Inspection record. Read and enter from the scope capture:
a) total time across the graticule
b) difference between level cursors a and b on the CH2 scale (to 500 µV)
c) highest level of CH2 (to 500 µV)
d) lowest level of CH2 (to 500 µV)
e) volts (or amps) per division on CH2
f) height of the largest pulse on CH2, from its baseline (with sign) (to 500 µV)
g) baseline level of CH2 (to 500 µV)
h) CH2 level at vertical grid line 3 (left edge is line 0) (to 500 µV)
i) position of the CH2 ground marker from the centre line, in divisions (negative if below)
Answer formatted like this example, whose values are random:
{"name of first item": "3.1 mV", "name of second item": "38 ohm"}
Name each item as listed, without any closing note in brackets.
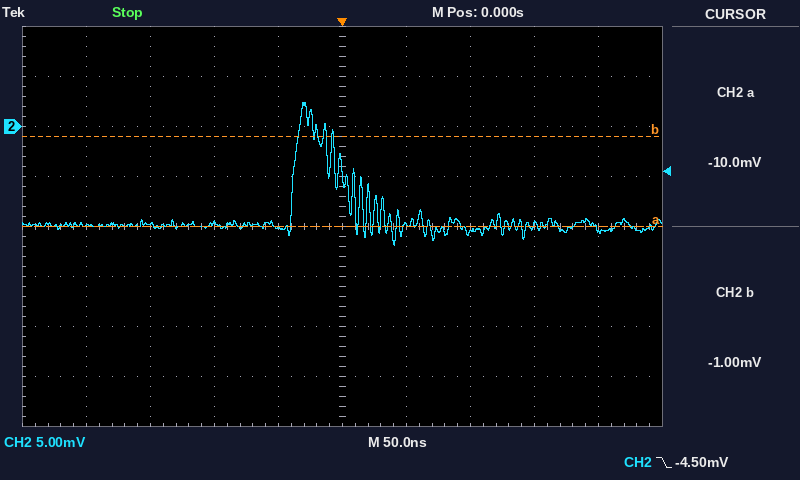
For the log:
{"total time across the graticule": "500 ns", "difference between level cursors a and b on the CH2 scale": "9.0 mV", "highest level of CH2": "2.5 mV", "lowest level of CH2": "-12.0 mV", "volts (or amps) per division on CH2": "5 mV", "height of the largest pulse on CH2, from its baseline (with sign)": "+12.5 mV", "baseline level of CH2": "-10.0 mV", "CH2 level at vertical grid line 3 (left edge is line 0)": "-9.5 mV", "position of the CH2 ground marker from the centre line, in divisions": "+2.0 div"}
